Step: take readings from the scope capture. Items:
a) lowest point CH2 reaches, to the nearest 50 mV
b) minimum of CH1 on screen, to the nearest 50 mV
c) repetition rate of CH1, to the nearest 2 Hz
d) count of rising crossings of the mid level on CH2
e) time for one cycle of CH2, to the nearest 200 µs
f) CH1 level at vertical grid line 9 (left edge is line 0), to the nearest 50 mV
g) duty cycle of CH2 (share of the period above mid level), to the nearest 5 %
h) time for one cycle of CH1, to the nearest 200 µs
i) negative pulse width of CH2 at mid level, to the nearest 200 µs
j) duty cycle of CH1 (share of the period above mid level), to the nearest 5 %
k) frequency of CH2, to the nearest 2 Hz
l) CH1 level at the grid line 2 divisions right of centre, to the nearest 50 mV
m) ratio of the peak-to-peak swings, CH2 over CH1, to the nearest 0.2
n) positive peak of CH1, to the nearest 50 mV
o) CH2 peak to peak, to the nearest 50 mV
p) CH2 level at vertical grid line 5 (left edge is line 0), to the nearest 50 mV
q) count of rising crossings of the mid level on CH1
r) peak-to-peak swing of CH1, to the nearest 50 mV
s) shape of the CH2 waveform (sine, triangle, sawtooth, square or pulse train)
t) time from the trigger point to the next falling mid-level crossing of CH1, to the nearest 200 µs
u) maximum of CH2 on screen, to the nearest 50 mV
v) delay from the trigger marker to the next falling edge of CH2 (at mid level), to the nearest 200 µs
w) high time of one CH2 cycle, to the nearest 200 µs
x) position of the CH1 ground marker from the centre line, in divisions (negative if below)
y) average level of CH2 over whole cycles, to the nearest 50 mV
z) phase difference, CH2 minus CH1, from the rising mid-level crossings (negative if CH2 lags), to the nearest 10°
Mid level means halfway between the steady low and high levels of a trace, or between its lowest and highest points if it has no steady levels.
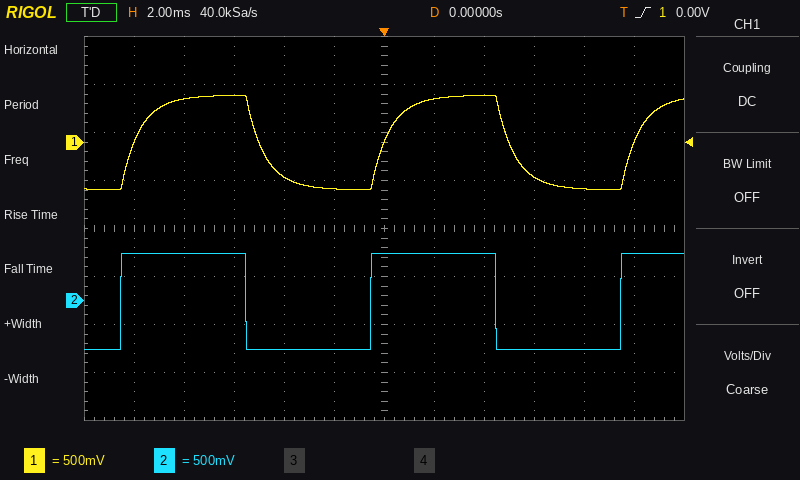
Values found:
-500 mV
-500 mV
100 Hz
3
10.0 ms
-350 mV
50 %
10.0 ms
5.0 ms
50 %
100 Hz
500 mV
1.0
500 mV
1.00 V
-500 mV
3
1.00 V
square
5.0 ms
500 mV
4.4 ms
5.0 ms
+1.8 div
0 mV
+20°
